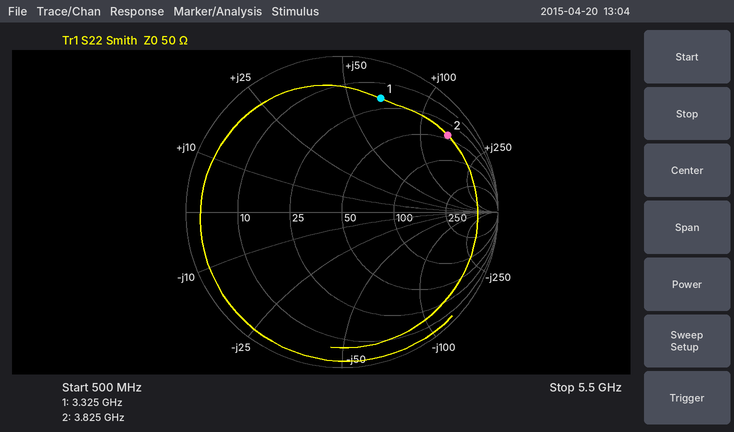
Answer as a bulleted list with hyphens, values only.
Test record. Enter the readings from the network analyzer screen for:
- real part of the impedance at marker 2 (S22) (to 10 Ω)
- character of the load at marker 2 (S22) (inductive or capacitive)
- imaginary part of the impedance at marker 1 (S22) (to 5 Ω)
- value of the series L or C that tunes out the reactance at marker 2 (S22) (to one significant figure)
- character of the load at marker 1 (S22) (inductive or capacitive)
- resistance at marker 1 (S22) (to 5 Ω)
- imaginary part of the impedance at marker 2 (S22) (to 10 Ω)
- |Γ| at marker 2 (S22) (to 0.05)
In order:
- 40 Ω
- inductive
- +65 Ω
- 300 fF
- inductive
- 20 Ω
- +140 Ω
- 0.85
